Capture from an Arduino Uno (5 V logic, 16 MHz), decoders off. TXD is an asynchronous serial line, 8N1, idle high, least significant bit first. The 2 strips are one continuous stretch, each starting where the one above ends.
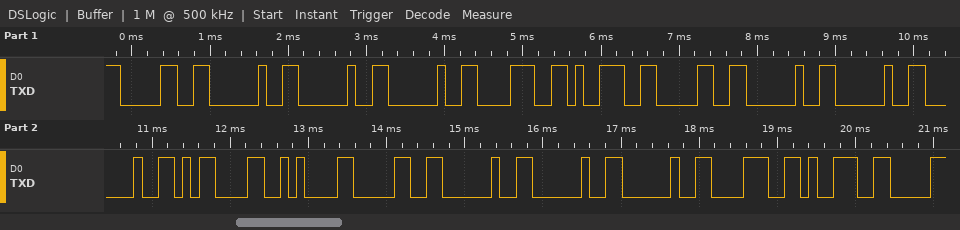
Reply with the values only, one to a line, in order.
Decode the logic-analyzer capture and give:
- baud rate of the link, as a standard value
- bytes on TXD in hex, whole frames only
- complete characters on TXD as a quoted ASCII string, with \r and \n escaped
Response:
9600 baud
30 20 20 20 38 39 30 20 20 20 0D 0A 30 20 20 20 38 39
"0   890   \r\n0   89"
